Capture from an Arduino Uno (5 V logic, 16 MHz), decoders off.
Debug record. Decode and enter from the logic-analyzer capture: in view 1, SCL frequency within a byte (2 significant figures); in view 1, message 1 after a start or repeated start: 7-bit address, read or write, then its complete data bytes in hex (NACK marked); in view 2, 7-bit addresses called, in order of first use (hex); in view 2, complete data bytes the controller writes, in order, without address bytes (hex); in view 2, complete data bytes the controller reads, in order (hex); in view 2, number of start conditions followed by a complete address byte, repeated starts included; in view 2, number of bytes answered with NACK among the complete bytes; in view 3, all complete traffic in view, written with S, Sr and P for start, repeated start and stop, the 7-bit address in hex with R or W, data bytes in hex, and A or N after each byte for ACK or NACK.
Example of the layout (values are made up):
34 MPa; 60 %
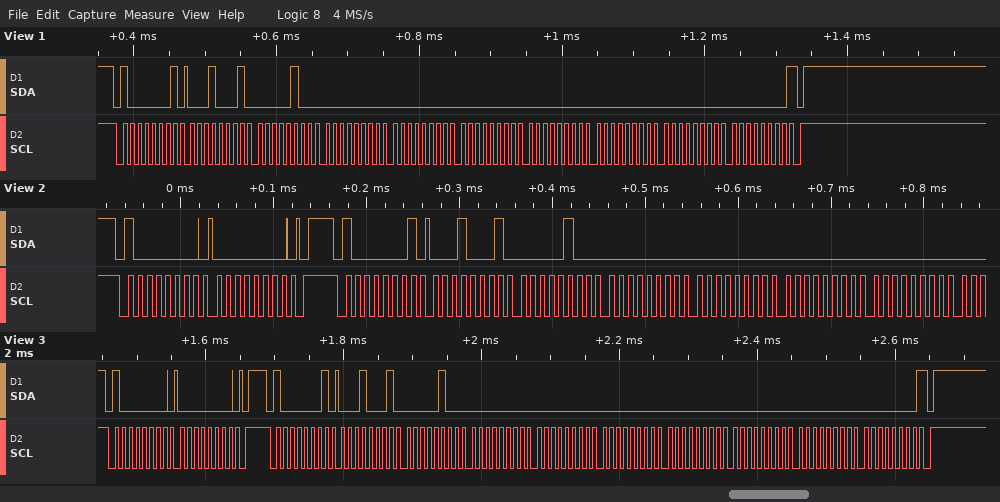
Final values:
100 kHz; 0x40 read: 11 04 00 00 00 00 00 00 00 NACK; 0x40; 00; 11 04 00 00 00 00; 2; 0; S 40W A 00 A P S 40R A 11 A 04 A 00 A 00 A 00 A 00 A 00 A 00 A 00 N P
